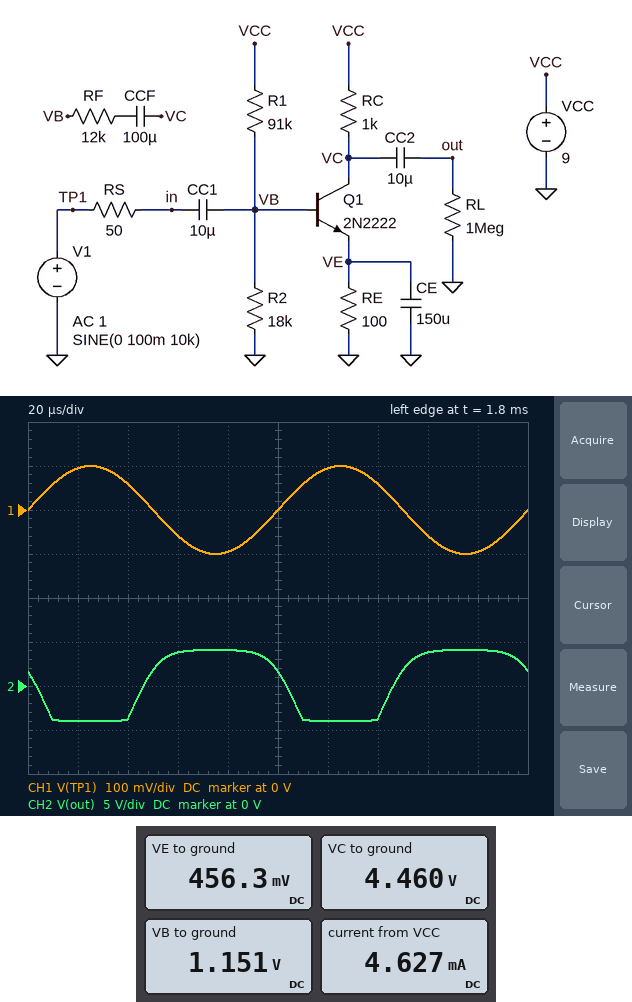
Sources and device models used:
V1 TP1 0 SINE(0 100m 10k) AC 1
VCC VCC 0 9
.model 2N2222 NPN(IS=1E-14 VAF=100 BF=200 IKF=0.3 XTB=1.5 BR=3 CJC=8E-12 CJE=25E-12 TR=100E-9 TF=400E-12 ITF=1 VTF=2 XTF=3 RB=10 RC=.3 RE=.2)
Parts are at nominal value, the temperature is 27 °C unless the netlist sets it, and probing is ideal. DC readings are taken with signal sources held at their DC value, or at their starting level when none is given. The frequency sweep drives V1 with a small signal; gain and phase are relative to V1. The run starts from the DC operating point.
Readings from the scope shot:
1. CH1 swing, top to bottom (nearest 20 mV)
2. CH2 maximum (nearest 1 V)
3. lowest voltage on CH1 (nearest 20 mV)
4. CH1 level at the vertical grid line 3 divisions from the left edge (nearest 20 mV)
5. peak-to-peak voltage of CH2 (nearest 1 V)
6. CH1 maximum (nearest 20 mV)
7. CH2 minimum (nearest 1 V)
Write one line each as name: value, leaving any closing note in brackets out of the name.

CH1 swing, top to bottom: 200 mV
CH2 maximum: 4 V
lowest voltage on CH1: -100 mV
CH1 level at the vertical grid line 3 divisions from the left edge: -60 mV
peak-to-peak voltage of CH2: 8 V
CH1 maximum: 100 mV
CH2 minimum: -4 V
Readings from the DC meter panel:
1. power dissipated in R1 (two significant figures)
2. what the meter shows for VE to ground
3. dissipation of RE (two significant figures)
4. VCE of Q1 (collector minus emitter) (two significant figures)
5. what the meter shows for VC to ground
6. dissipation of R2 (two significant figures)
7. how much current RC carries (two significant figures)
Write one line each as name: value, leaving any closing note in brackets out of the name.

power dissipated in R1: 680 µW
what the meter shows for VE to ground: 456.3 mV
dissipation of RE: 2.1 mW
VCE of Q1 (collector minus emitter): 4.0 V
what the meter shows for VC to ground: 4.460 V
dissipation of R2: 74 µW
how much current RC carries: 4.5 mA
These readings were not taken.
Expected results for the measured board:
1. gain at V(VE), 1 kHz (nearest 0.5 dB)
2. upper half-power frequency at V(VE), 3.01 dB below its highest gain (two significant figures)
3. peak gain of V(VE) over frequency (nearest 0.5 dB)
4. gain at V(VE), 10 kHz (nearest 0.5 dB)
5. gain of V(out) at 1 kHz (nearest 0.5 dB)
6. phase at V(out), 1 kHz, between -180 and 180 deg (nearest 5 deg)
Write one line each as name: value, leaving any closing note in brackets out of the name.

gain at V(VE), 1 kHz: -20.0 dB
upper half-power frequency at V(VE), 3.01 dB below its highest gain: 250 Hz
peak gain of V(VE) over frequency: -7.5 dB
gain at V(VE), 10 kHz: -40.0 dB
gain of V(out) at 1 kHz: 38.5 dB
phase at V(out), 1 kHz, between -180 and 180 deg: -165 deg
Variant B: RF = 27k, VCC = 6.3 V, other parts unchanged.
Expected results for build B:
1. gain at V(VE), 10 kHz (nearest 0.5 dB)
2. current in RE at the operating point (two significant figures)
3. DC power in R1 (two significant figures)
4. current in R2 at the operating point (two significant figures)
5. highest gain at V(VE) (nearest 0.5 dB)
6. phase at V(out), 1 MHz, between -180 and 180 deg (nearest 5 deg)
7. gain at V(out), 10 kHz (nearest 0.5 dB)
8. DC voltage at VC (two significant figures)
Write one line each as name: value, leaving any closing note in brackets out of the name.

gain at V(VE), 10 kHz: -43.0 dB
current in RE at the operating point: 2.1 mA
DC power in R1: 320 µW
current in R2 at the operating point: 49 µA
highest gain at V(VE): -5.0 dB
phase at V(out), 1 MHz, between -180 and 180 deg: 170 deg
gain at V(out), 10 kHz: 36.0 dB
DC voltage at VC: 4.2 V
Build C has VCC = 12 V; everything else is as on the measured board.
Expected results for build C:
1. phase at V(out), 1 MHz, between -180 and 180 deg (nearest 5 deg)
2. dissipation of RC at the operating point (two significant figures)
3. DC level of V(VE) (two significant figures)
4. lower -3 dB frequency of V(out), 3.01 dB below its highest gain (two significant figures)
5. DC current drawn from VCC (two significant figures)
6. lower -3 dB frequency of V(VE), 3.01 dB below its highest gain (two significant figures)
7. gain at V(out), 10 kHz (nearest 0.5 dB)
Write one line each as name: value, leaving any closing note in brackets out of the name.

phase at V(out), 1 MHz, between -180 and 180 deg: 165 deg
dissipation of RC at the operating point: 53 mW
DC level of V(VE): 730 mV
lower -3 dB frequency of V(out), 3.01 dB below its highest gain: 290 Hz
DC current drawn from VCC: 7.4 mA
lower -3 dB frequency of V(VE), 3.01 dB below its highest gain: 6.5 Hz
gain at V(out), 10 kHz: 41.0 dB
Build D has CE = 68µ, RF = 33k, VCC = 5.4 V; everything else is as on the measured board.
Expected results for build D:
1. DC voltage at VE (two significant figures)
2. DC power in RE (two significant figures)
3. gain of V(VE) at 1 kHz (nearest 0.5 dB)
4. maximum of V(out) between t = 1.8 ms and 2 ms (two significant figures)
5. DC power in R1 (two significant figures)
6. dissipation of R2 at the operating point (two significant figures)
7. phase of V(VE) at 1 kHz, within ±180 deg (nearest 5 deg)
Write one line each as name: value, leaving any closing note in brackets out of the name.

DC voltage at VE: 130 mV
DC power in RE: 180 µW
gain of V(VE) at 1 kHz: -19.5 dB
maximum of V(out) between t = 1.8 ms and 2 ms: 1.3 V
DC power in R1: 230 µW
dissipation of R2 at the operating point: 35 µW
phase of V(VE) at 1 kHz, within ±180 deg: -80 deg
